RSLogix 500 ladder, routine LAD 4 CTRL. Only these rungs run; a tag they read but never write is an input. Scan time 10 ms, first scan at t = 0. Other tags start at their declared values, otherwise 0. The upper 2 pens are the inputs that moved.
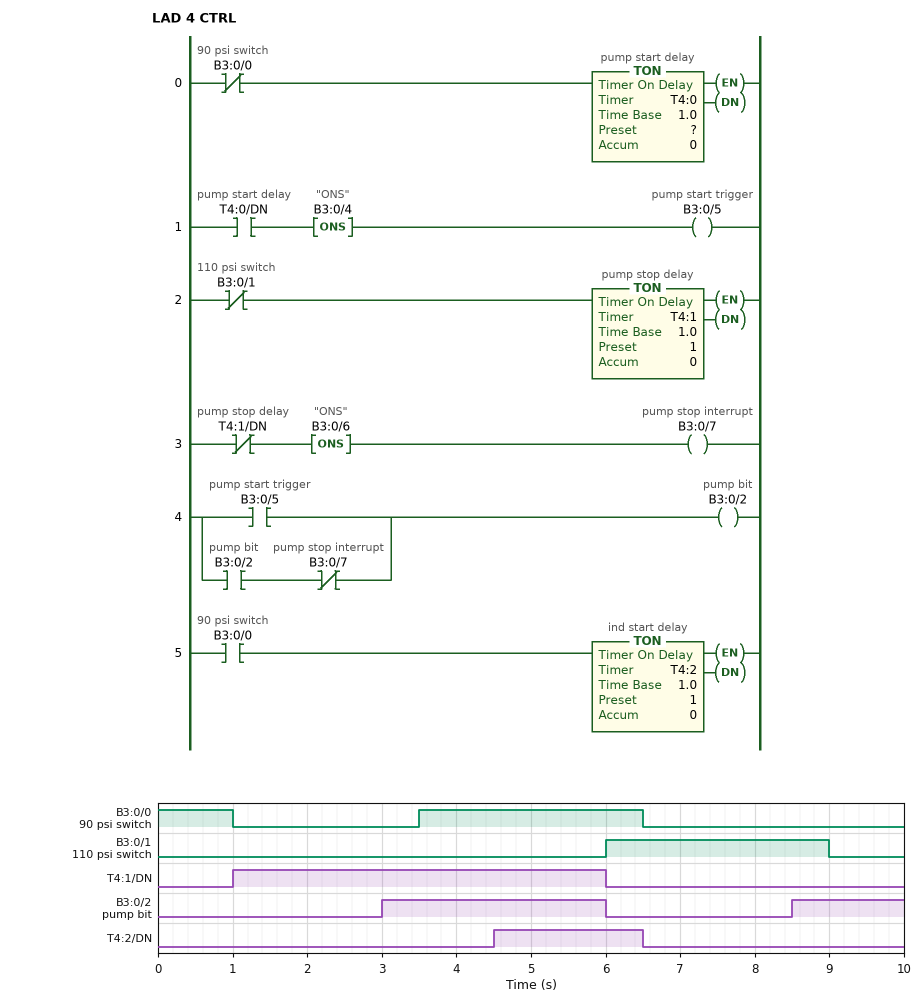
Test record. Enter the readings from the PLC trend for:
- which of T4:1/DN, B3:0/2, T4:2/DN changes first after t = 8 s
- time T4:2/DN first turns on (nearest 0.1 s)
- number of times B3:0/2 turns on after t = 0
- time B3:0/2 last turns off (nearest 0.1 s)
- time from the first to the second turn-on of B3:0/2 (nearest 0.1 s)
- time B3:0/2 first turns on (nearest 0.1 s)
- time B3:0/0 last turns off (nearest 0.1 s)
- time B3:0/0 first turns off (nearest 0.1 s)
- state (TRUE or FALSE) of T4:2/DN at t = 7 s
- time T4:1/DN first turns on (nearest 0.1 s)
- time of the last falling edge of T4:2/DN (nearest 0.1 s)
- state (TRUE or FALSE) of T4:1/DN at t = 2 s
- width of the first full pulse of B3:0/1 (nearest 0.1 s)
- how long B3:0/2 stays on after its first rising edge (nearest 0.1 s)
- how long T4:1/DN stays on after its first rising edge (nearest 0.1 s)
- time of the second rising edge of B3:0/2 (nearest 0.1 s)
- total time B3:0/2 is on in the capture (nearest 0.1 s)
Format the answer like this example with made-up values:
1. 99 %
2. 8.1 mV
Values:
1. B3:0/2
2. 4.5 s
3. 2
4. 6.0 s
5. 5.5 s
6. 3.0 s
7. 6.5 s
8. 1.0 s
9. FALSE
10. 1.0 s
11. 6.5 s
12. TRUE
13. 3.0 s
14. 3.0 s
15. 5.0 s
16. 8.5 s
17. 4.5 s
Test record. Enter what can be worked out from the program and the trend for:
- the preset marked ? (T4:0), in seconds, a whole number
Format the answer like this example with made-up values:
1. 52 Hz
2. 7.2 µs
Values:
1. 2 s
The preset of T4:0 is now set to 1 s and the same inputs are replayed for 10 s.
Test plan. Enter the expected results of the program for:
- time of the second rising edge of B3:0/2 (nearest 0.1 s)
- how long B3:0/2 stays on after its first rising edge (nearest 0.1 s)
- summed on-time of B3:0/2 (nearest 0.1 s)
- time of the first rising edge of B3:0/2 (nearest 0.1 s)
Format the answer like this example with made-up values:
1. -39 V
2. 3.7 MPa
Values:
1. 7.5 s
2. 4.0 s
3. 6.5 s
4. 2.0 s
